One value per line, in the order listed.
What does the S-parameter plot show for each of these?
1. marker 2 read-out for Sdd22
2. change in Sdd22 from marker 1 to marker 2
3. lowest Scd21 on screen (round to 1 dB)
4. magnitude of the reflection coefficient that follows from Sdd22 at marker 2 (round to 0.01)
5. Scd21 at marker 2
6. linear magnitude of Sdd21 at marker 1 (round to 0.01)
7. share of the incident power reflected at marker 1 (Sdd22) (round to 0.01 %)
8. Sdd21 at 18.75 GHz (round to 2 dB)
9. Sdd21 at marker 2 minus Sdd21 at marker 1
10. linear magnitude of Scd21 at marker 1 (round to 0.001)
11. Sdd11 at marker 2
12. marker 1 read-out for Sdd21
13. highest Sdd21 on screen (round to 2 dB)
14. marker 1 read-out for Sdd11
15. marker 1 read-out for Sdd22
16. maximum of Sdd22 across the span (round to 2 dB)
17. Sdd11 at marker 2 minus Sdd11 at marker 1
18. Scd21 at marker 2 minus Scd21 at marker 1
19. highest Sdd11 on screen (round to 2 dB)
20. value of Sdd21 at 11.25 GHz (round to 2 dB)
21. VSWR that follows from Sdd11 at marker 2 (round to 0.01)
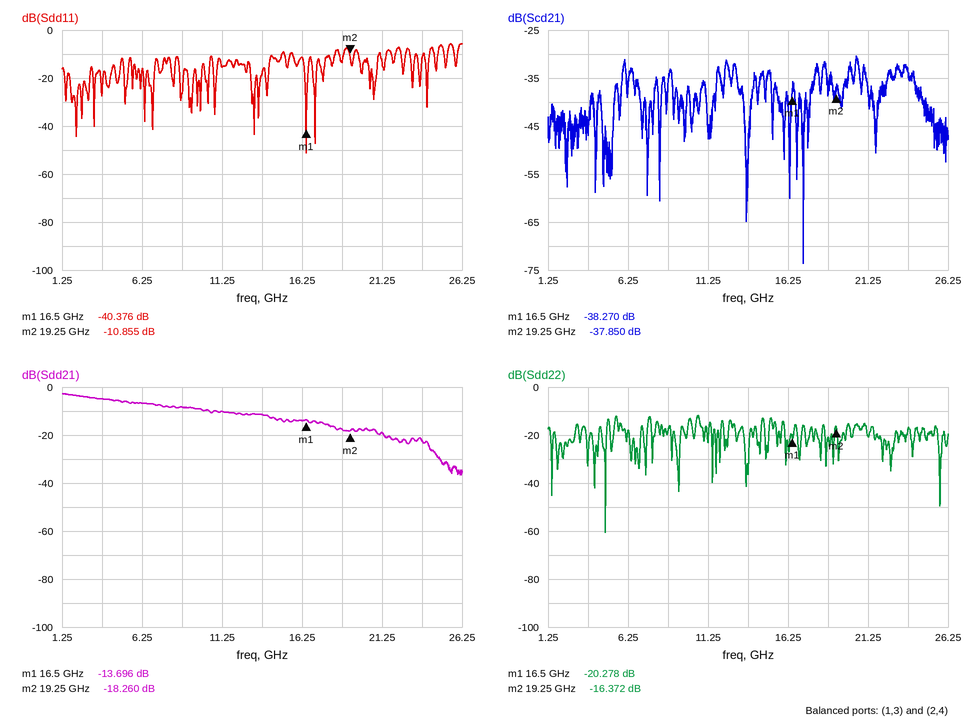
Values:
-16.372 dB
3.906 dB
-74 dB
0.15
-37.850 dB
0.21
0.94 %
-18 dB
-4.564 dB
0.012
-10.855 dB
-13.696 dB
-2 dB
-40.376 dB
-20.278 dB
-12 dB
29.521 dB
0.420 dB
-6 dB
-10 dB
1.80
